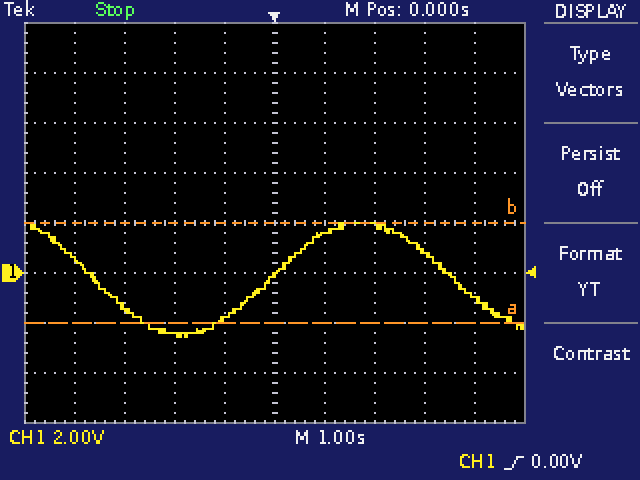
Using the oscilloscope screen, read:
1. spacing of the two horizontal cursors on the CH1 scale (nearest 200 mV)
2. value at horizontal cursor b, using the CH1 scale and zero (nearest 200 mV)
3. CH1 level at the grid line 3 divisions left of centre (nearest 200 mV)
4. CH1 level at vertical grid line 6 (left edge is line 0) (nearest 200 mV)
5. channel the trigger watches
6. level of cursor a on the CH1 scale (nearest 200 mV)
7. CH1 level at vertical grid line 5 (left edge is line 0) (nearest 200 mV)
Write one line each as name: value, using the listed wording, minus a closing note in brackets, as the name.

spacing of the two horizontal cursors on the CH1 scale: 4.0 V
value at horizontal cursor b, using the CH1 scale and zero: 2.0 V
CH1 level at the grid line 3 divisions left of centre: -1.4 V
CH1 level at vertical grid line 6 (left edge is line 0): 1.6 V
channel the trigger watches: CH1
level of cursor a on the CH1 scale: -2.0 V
CH1 level at vertical grid line 5 (left edge is line 0): 0.0 V
